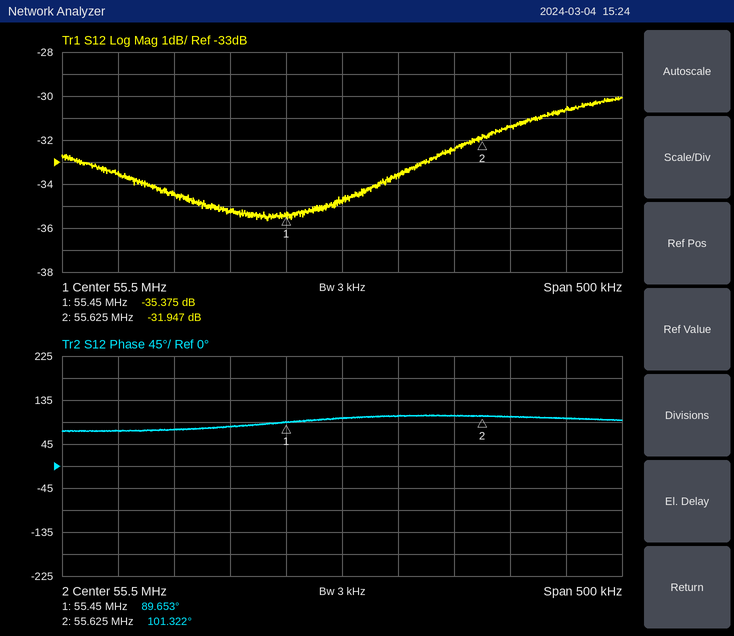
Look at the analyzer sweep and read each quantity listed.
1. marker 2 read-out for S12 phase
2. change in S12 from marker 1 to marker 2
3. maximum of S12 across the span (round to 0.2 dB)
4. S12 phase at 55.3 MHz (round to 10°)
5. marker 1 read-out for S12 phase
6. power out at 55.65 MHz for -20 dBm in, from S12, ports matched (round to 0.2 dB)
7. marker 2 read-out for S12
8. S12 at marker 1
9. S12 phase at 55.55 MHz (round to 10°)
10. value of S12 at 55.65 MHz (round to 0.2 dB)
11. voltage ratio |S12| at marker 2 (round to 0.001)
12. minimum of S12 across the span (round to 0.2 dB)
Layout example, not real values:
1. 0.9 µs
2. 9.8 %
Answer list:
1. 101.322°
2. 3.428 dB
3. -30.0 dB
4. 70°
5. 89.653°
6. -51.4 dBm
7. -31.947 dB
8. -35.375 dB
9. 100°
10. -31.4 dB
11. 0.025
12. -35.6 dB
